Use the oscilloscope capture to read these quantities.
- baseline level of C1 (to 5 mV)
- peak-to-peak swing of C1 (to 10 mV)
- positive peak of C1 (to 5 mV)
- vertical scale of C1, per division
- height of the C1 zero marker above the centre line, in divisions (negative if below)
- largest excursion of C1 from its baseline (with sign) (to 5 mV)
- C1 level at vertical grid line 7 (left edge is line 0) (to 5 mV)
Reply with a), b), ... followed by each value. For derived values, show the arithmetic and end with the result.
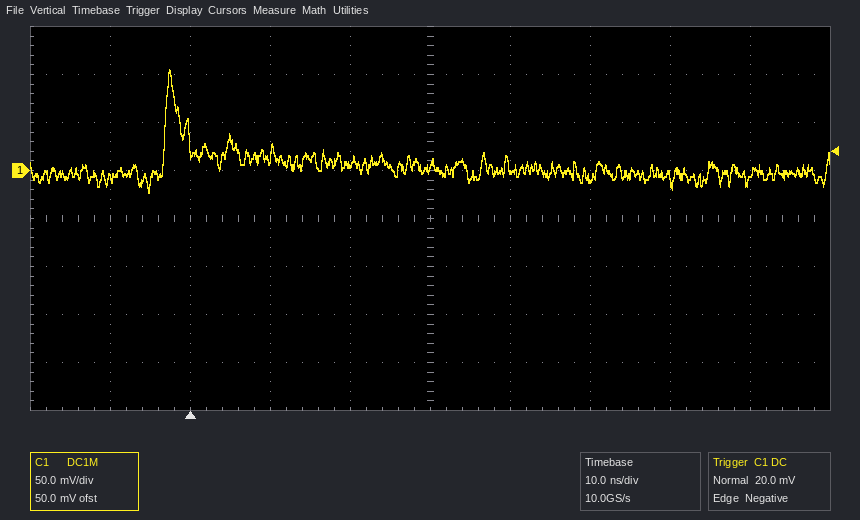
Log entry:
a) 0 mV
b) 130 mV
c) 105 mV
d) 50 mV
e) +1.0 div
f) 105 mV − (0 mV) = +105 mV
g) -10 mV
